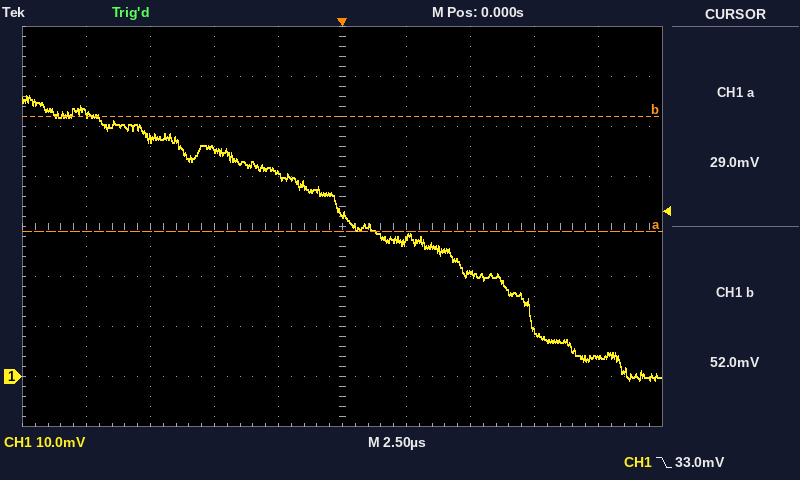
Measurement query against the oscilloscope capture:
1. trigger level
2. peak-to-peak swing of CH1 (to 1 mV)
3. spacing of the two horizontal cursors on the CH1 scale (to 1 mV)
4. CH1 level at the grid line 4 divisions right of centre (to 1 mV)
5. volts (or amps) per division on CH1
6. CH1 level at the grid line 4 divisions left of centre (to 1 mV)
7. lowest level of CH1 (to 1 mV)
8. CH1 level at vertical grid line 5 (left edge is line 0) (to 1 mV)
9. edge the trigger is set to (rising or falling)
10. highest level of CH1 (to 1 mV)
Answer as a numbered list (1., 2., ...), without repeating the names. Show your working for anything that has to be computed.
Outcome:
1. 33.0 mV
2. 56 mV − (-1 mV) = 57 mV
3. 23 mV
4. 4 mV
5. 10 mV
6. 53 mV
7. -1 mV
8. 33 mV
9. falling
10. 56 mV
